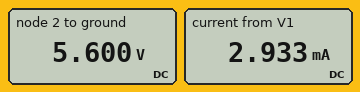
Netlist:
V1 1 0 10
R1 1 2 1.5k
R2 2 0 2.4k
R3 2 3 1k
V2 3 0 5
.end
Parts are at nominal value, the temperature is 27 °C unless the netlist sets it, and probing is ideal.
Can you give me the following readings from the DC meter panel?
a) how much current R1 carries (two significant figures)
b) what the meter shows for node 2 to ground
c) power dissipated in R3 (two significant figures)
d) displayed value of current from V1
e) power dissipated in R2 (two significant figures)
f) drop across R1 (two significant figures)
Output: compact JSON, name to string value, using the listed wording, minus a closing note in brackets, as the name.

{"how much current R1 carries": "2.9 mA", "what the meter shows for node 2 to ground": "5.600 V", "power dissipated in R3": "360 µW", "displayed value of current from V1": "2.933 mA", "power dissipated in R2": "13 mW", "drop across R1": "4.4 V"}
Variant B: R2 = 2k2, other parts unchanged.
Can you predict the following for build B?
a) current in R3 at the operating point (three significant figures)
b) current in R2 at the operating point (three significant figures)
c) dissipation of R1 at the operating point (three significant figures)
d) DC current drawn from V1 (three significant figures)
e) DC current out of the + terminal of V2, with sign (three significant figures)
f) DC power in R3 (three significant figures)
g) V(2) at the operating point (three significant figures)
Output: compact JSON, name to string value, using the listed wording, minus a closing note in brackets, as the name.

{"current in R3 at the operating point": "500 µA", "current in R2 at the operating point": "2.50 mA", "dissipation of R1 at the operating point": "13.5 mW", "DC current drawn from V1": "3.00 mA", "DC current out of the + terminal of V2, with sign": "-500 µA", "DC power in R3": "250 µW", "V(2) at the operating point": "5.50 V"}
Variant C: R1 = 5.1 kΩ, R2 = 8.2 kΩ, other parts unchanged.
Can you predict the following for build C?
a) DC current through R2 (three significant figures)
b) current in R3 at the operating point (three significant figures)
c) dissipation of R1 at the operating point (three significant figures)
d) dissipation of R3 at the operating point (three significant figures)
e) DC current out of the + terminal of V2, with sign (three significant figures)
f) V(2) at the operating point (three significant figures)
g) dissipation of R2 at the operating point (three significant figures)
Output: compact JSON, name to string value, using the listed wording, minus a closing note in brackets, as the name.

{"DC current through R2": "644 µA", "current in R3 at the operating point": "281 µA", "dissipation of R1 at the operating point": "4.37 mW", "dissipation of R3 at the operating point": "79.1 µW", "DC current out of the + terminal of V2, with sign": "-281 µA", "V(2) at the operating point": "5.28 V", "dissipation of R2 at the operating point": "3.40 mW"}
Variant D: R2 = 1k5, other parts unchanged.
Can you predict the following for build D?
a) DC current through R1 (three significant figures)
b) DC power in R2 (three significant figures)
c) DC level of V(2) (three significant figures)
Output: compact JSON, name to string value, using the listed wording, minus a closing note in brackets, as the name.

{"DC current through R1": "3.33 mA", "DC power in R2": "16.7 mW", "DC level of V(2)": "5.00 V"}
